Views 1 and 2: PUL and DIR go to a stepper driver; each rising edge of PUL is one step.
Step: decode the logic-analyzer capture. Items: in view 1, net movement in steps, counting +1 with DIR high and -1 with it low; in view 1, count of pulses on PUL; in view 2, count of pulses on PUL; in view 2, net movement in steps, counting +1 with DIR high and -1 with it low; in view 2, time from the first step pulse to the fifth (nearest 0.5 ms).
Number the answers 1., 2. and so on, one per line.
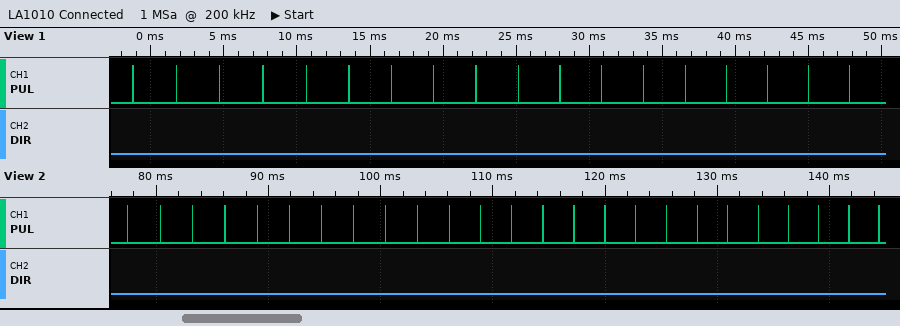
1. -18
2. 18
3. 25
4. -25
5. 11.5 ms
